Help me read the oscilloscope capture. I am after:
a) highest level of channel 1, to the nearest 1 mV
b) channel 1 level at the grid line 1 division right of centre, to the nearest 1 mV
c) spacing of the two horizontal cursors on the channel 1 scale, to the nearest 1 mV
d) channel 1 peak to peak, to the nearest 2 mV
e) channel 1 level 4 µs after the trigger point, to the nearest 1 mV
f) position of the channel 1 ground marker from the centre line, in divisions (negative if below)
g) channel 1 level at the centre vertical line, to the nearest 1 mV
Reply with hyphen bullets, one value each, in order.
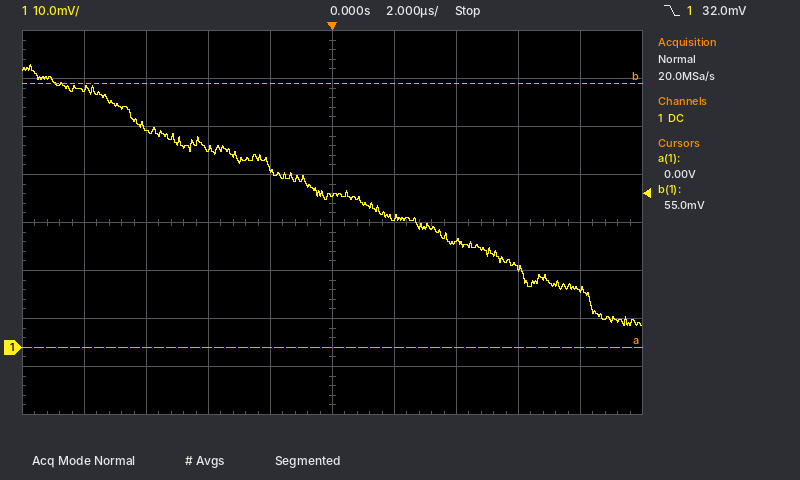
- 59 mV
- 27 mV
- 55 mV
- 54 mV
- 22 mV
- -2.6 div
- 32 mV
